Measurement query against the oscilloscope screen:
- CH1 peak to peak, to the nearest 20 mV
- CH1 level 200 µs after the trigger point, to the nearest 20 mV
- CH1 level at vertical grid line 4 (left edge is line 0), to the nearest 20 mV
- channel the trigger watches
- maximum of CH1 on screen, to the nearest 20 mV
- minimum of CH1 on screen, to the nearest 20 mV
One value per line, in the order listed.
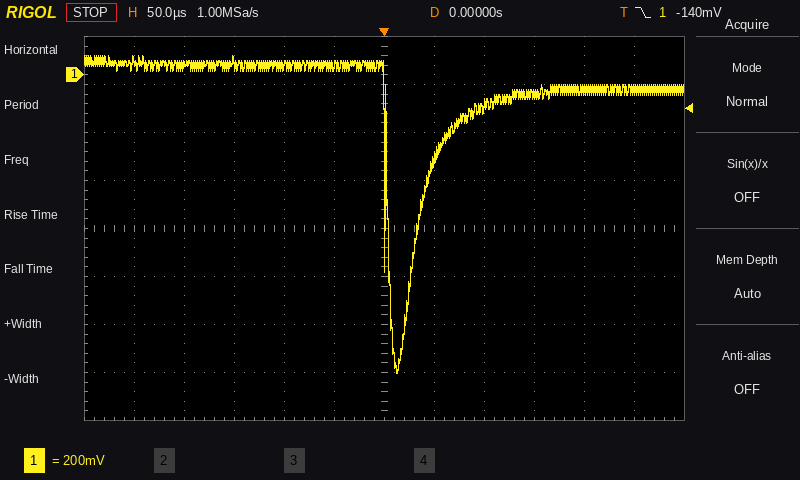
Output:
1.32 V
-60 mV
40 mV
CH1
80 mV
-1.24 V
